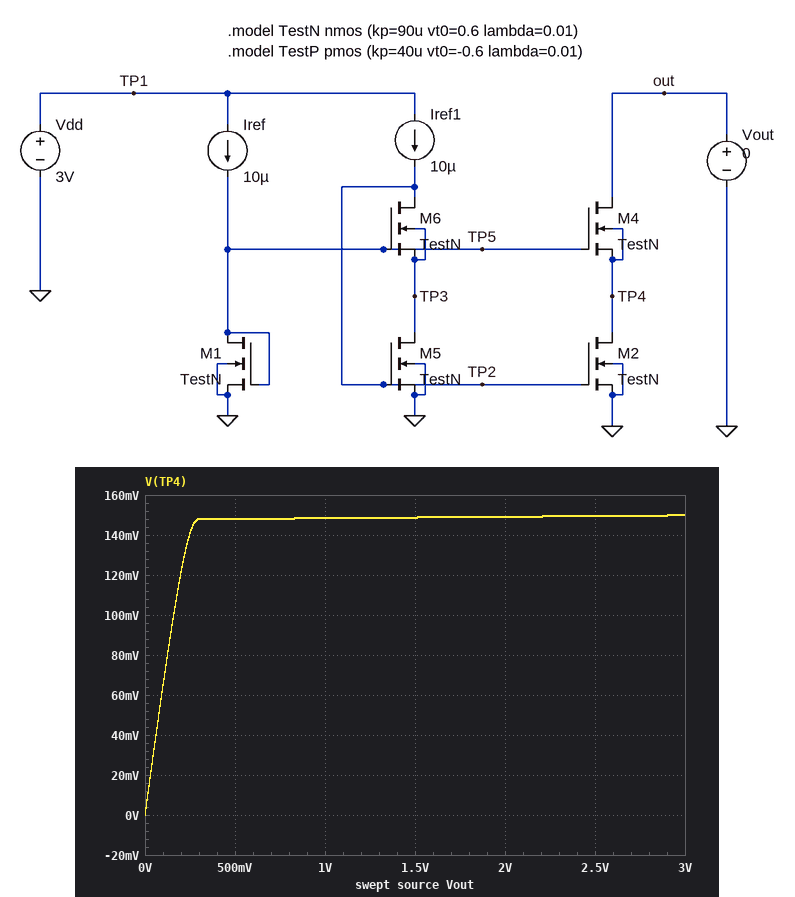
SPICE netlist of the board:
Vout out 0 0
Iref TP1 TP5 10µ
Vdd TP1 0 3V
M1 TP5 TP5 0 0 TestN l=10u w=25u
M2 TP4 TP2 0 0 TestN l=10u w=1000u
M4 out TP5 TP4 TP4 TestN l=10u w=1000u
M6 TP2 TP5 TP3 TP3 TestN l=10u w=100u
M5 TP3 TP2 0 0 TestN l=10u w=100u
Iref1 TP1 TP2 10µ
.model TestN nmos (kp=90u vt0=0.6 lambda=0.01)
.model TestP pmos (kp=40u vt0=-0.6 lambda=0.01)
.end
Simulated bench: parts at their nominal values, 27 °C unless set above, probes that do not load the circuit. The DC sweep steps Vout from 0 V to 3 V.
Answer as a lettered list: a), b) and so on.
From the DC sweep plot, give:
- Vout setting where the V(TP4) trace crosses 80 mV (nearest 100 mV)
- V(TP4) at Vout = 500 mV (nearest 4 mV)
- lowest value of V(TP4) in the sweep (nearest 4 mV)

a) 100 mV
b) 148 mV
c) 0 V
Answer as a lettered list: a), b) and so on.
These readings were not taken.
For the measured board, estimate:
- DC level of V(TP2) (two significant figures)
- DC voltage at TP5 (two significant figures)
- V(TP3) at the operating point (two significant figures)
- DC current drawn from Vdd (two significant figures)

a) 750 mV
b) 900 mV
c) 150 mV
d) 20 µA
